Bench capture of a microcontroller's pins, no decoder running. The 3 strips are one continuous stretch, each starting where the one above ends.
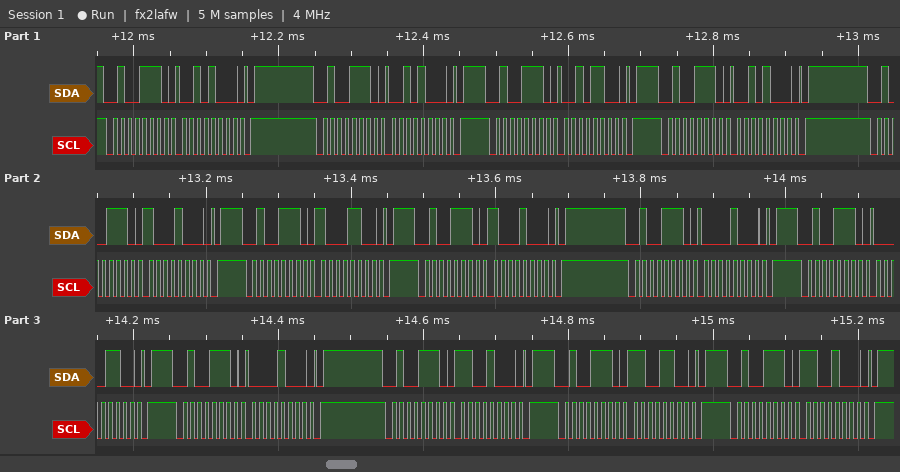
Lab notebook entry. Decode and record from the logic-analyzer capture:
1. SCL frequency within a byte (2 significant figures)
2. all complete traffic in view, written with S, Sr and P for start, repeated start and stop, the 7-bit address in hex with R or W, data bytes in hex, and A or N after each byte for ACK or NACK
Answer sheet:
100 kHz
S 27W A 28 A P S 27W A 28 A P S 27W A 2C A P S 27W A 28 A P S 27W A 88 A P S 27W A 8C A P S 27W A 88 A P S 27W A 08 A P S 27W A 0C A P S 27W A 08 A P S 27W A C8 A P S 27W A CC A P S 27W A C8 A P
